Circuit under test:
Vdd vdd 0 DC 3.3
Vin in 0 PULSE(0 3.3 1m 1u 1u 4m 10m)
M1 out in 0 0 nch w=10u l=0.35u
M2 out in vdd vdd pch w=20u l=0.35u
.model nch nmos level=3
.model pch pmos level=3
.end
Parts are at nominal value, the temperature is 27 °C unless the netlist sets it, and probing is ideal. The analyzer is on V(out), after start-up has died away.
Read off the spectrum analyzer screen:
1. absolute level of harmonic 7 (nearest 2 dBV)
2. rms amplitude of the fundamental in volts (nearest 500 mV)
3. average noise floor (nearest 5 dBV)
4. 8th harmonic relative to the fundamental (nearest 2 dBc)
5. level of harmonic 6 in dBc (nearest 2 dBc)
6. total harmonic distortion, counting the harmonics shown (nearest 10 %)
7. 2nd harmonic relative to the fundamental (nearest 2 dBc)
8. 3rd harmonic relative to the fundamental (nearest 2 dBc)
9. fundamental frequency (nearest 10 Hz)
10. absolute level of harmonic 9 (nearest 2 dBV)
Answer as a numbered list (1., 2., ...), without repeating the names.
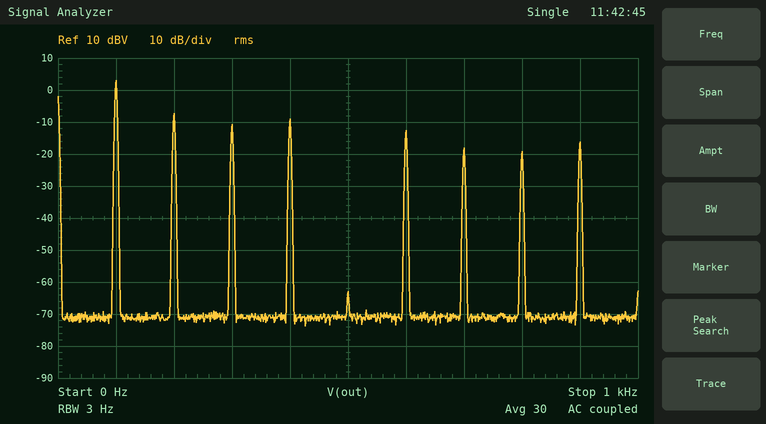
1. -18 dBV
2. 1.5 V
3. -70 dBV
4. -22 dBc
5. -16 dBc
6. 50 %
7. -10 dBc
8. -14 dBc
9. 100 Hz
10. -16 dBV
